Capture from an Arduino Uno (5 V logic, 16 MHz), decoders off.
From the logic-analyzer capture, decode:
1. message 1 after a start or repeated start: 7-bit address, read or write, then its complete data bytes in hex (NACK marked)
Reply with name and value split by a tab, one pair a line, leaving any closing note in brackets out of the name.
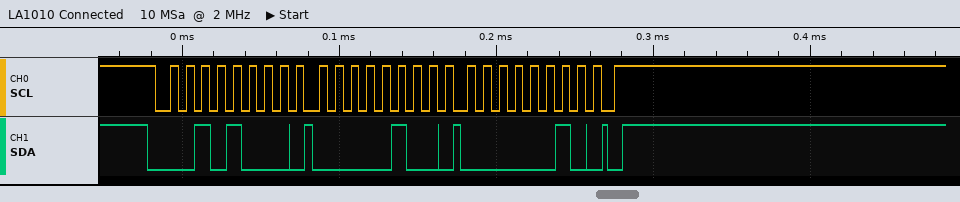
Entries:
message 1 after a start or repeated start: 7-bit address, read or write, then its complete data bytes in hex	0x14 write: 04 02
